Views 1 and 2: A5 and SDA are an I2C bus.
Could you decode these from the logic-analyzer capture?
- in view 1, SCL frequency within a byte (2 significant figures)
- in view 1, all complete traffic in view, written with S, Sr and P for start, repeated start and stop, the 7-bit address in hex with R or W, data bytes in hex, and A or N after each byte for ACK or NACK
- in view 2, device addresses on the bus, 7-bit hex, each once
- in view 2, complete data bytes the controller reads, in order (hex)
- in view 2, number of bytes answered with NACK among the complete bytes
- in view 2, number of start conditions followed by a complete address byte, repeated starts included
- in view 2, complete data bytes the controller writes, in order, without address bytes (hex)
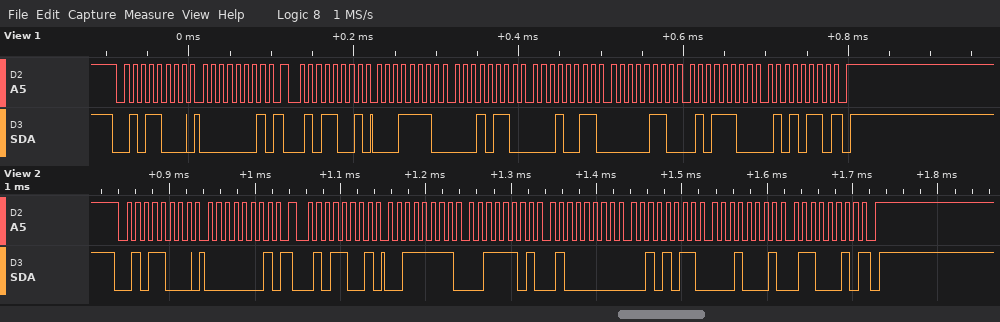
100 kHz
S 2CW A 01 A Sr 2CR A 1E A 16 A 13 A 06 A 5C A 56 N P
0x2C
3F 3D 40 2B 11 62
1
2
01
